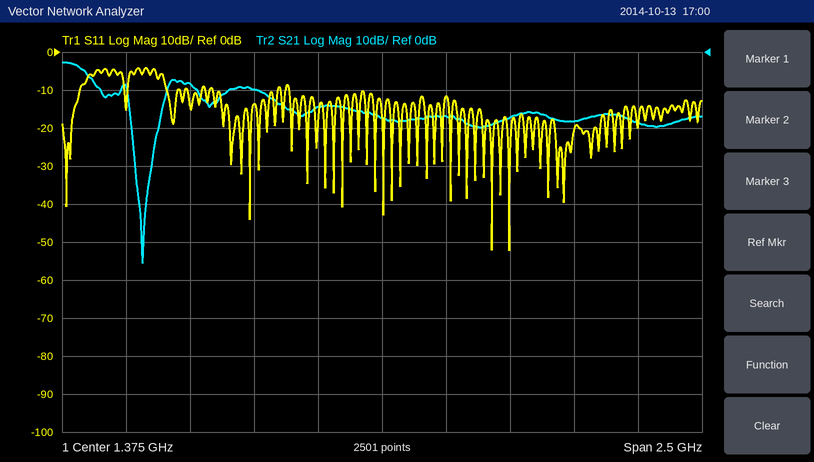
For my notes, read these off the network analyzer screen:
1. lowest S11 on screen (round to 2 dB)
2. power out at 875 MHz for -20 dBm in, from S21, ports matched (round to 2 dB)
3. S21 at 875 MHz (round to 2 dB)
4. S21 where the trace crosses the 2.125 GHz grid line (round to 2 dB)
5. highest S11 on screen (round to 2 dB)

-52 dB
-30 dBm
-10 dB
-18 dB
-4 dB
